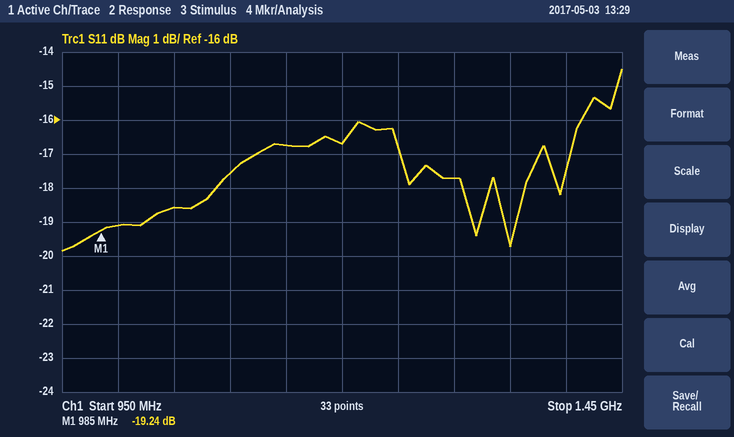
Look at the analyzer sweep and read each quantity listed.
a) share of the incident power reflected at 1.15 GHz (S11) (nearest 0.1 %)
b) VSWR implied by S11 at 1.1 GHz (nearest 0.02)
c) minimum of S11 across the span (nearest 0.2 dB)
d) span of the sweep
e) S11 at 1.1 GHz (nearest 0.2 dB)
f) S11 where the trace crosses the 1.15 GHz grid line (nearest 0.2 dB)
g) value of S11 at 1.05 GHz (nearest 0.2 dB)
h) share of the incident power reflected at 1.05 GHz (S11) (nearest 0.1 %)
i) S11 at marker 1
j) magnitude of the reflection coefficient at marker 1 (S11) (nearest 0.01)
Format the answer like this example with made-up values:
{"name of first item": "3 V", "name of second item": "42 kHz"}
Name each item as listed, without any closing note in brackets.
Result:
{"share of the incident power reflected at 1.15 GHz (S11)": "2.1 %", "VSWR implied by S11 at 1.1 GHz": "1.30", "minimum of S11 across the span": "-19.8 dB", "span of the sweep": "500 MHz", "S11 at 1.1 GHz": "-17.6 dB", "S11 where the trace crosses the 1.15 GHz grid line": "-16.8 dB", "value of S11 at 1.05 GHz": "-18.6 dB", "share of the incident power reflected at 1.05 GHz (S11)": "1.4 %", "S11 at marker 1": "-19.24 dB", "magnitude of the reflection coefficient at marker 1 (S11)": "0.11"}
